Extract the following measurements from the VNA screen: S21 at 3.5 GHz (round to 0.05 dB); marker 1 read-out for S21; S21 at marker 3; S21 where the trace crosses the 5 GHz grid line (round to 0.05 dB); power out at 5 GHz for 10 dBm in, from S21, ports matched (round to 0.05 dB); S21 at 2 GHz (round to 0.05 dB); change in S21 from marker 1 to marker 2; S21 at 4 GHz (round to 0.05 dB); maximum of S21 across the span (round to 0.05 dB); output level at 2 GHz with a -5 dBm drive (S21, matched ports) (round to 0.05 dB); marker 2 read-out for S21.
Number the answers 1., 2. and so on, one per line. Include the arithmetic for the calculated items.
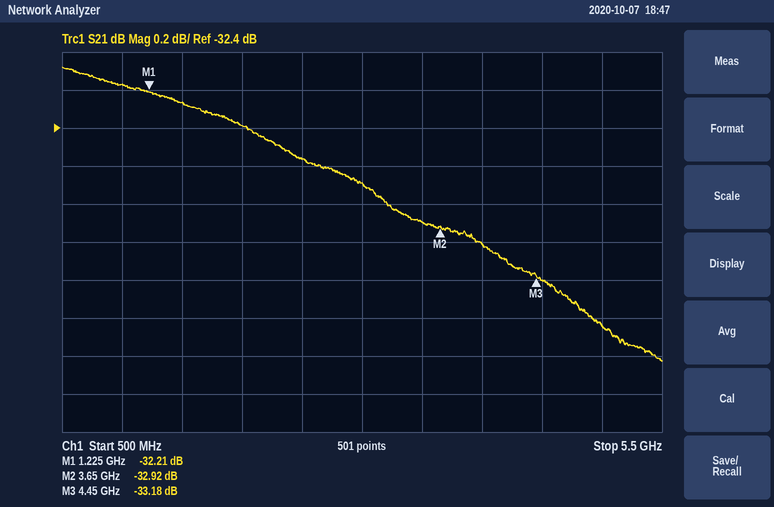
1. -32.90 dB
2. -32.21 dB
3. -33.18 dB
4. -33.45 dB
5. 10 dBm + (-33.45 dB) = -23.45 dBm
6. -32.40 dB
7. -32.92 − (-32.21) = -0.71 dB
8. -33.00 dB
9. -32.10 dB
10. -5 dBm + (-32.40 dB) = -37.40 dBm
11. -32.92 dB
